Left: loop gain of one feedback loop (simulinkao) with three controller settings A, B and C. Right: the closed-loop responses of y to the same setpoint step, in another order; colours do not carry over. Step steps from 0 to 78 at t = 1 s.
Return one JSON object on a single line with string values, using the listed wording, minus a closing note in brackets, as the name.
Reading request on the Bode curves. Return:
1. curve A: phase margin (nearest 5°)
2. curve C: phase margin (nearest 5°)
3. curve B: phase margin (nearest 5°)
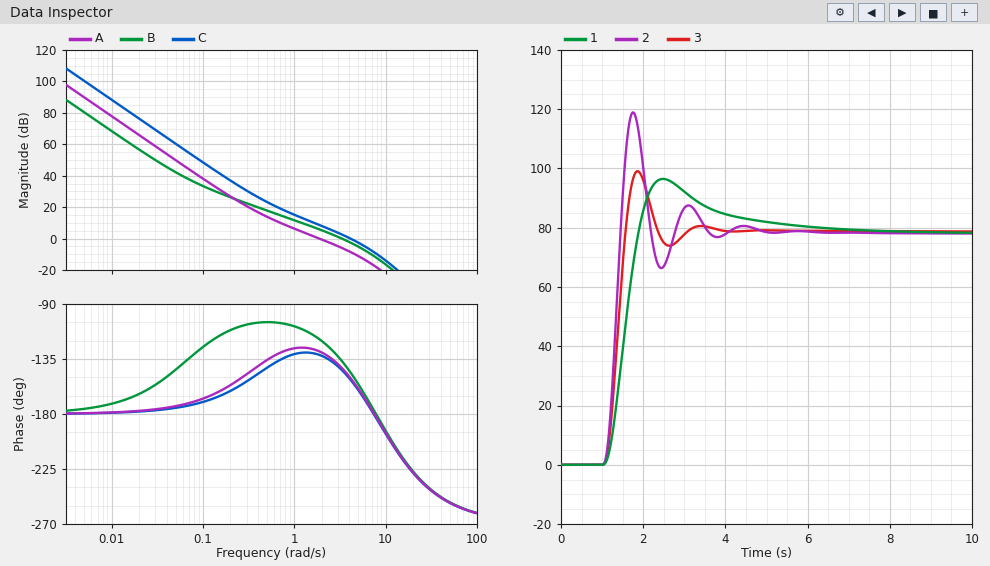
{"curve A: phase margin": "50°", "curve C: phase margin": "30°", "curve B: phase margin": "45°"}
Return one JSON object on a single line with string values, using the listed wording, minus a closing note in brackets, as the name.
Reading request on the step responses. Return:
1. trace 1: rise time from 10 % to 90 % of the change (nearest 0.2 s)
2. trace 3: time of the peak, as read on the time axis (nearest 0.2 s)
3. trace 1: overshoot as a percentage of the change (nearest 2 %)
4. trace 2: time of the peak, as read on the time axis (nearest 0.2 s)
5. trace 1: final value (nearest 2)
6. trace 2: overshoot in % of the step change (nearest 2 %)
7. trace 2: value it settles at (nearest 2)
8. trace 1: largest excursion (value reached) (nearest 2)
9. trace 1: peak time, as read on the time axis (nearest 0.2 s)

{"trace 1: rise time from 10 % to 90 % of the change": "0.6 s", "trace 3: time of the peak, as read on the time axis": "1.8 s", "trace 1: overshoot as a percentage of the change": "24 %", "trace 2: time of the peak, as read on the time axis": "1.8 s", "trace 1: final value": "78", "trace 2: overshoot in % of the step change": "52 %", "trace 2: value it settles at": "78", "trace 1: largest excursion (value reached)": "96", "trace 1: peak time, as read on the time axis": "2.4 s"}
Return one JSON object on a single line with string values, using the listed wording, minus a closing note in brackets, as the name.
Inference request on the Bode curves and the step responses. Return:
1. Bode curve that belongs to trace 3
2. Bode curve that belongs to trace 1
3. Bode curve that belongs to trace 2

{"Bode curve that belongs to trace 3": "B", "Bode curve that belongs to trace 1": "A", "Bode curve that belongs to trace 2": "C"}
